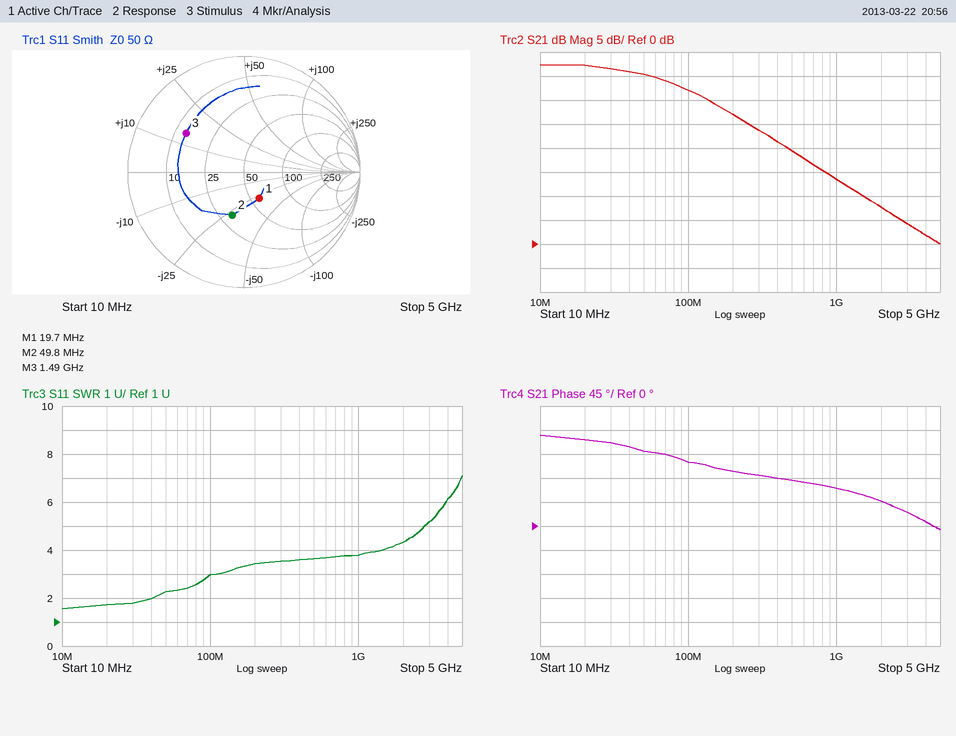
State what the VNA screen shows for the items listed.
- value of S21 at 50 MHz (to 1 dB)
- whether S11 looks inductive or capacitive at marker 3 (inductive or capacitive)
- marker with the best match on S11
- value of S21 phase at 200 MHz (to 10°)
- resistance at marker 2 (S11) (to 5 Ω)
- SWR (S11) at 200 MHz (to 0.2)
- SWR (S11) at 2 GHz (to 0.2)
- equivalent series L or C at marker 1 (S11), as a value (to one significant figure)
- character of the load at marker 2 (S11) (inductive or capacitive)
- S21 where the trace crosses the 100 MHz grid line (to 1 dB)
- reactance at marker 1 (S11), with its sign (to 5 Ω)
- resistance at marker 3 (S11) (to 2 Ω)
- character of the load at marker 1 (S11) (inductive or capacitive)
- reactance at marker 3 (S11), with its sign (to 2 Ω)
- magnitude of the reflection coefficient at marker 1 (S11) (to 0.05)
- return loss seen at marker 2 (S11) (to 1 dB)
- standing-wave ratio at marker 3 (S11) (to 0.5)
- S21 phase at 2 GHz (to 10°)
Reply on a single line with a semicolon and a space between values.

35 dB; inductive; marker 1; 100°; 30 Ω; 3.4; 4.4; 300 pF; capacitive; 32 dB; -30 Ω; 14 Ω; capacitive; +14 Ω; 0.25; 8 dB; 4.0; 50°
